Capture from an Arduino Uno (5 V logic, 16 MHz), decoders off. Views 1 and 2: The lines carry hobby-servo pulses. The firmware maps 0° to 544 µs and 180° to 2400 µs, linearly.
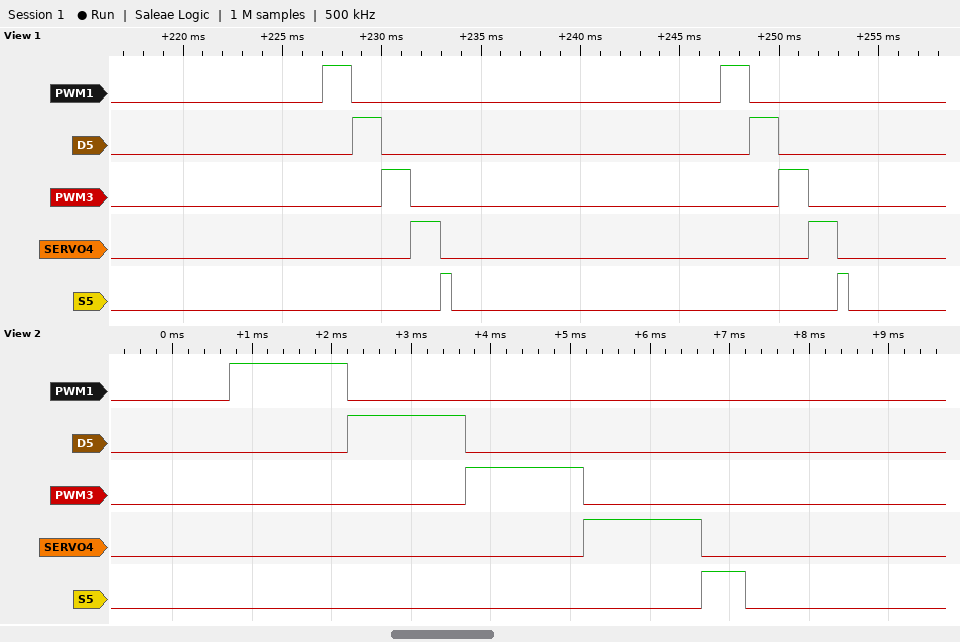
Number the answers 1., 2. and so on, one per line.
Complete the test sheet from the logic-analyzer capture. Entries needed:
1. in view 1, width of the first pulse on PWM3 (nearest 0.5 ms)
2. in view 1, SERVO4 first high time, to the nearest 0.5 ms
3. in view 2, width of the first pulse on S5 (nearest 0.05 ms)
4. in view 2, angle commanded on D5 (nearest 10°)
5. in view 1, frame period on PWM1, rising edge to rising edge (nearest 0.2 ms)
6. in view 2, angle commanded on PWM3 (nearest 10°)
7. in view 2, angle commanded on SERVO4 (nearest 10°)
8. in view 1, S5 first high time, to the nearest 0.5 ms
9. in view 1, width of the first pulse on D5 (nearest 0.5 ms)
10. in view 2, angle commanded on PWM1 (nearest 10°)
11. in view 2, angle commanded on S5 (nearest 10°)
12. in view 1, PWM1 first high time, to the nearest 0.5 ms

1. 1.5 ms
2. 1.5 ms
3. 0.55 ms
4. 90°
5. 20.0 ms
6. 90°
7. 90°
8. 0.5 ms
9. 1.5 ms
10. 90°
11. 0°
12. 1.5 ms
